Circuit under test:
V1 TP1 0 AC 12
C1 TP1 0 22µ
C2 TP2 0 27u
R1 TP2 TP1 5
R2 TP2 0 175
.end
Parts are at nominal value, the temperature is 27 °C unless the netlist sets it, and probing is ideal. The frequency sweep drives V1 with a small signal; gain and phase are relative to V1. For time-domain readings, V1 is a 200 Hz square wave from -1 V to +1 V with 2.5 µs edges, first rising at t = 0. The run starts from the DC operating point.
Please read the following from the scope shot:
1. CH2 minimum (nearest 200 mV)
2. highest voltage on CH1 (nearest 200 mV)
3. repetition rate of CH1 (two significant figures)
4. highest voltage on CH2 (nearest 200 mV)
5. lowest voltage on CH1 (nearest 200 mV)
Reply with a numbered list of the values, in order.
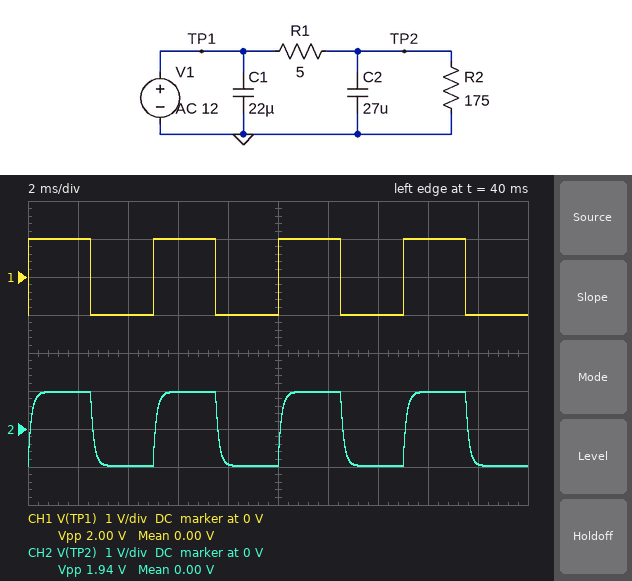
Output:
1. -1.0 V
2. 1.0 V
3. 200 Hz
4. 1.0 V
5. -1.0 V
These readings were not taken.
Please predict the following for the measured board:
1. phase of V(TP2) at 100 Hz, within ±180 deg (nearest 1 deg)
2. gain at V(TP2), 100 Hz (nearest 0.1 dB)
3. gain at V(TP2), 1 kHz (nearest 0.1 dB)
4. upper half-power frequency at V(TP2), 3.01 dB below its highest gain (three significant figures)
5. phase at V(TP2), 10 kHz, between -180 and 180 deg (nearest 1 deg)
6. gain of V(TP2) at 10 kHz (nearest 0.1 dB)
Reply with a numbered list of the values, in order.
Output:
1. -5 deg
2. -0.3 dB
3. -2.5 dB
4. 1.21 kHz
5. -83 deg
6. -18.6 dB
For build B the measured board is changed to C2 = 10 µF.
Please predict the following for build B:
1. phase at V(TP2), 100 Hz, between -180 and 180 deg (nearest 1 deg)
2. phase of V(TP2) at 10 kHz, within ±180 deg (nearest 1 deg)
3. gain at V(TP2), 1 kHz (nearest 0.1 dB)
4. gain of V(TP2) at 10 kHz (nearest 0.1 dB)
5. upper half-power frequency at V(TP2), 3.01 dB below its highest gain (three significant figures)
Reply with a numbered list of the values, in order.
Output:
1. -2 deg
2. -72 deg
3. -0.6 dB
4. -10.4 dB
5. 3.27 kHz
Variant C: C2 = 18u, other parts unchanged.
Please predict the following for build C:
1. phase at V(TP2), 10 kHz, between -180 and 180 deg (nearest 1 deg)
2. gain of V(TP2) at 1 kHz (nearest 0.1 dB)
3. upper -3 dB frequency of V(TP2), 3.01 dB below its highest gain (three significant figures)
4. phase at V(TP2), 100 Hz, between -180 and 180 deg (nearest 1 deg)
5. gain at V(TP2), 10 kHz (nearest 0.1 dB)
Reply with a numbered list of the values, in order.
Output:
1. -80 deg
2. -1.4 dB
3. 1.82 kHz
4. -3 deg
5. -15.2 dB
